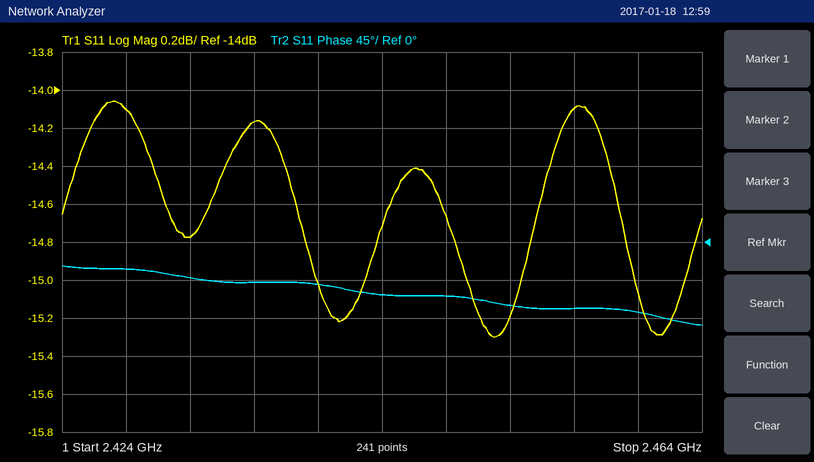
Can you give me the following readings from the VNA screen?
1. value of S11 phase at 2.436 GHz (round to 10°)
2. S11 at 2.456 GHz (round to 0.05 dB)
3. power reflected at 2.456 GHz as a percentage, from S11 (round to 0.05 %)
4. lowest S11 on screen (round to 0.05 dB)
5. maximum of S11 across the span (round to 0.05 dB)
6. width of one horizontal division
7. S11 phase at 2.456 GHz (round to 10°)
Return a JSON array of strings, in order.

["-50°", "-14.10 dB", "3.90 %", "-15.30 dB", "-14.05 dB", "4 MHz", "-80°"]
